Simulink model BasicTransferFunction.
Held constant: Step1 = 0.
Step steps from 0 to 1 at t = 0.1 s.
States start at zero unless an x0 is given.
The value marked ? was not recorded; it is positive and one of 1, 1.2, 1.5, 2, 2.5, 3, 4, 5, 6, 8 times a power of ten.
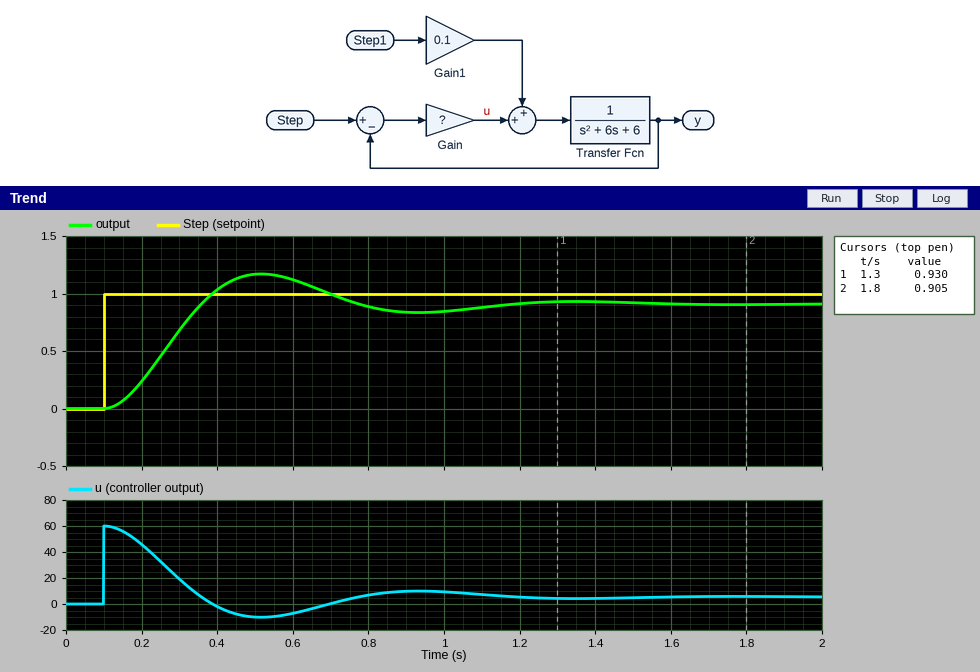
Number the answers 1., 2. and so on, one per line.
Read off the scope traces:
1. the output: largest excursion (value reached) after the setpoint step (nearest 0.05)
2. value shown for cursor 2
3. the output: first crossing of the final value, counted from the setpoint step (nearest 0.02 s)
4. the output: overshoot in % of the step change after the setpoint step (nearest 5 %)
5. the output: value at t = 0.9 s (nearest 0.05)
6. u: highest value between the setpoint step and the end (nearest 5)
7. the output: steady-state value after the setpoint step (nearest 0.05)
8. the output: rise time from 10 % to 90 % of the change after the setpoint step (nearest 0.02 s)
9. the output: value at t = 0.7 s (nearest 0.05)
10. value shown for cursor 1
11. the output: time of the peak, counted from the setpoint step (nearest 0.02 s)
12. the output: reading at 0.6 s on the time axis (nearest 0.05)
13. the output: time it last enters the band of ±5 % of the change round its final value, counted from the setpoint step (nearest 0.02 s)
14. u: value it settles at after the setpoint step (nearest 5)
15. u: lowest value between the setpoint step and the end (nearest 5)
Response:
1. 1.15
2. 0.905
3. 0.26 s
4. 30 %
5. 0.85
6. 60
7. 0.90
8. 0.18 s
9. 1.00
10. 0.930
11. 0.42 s
12. 1.10
13. 0.96 s
14. 5
15. -10
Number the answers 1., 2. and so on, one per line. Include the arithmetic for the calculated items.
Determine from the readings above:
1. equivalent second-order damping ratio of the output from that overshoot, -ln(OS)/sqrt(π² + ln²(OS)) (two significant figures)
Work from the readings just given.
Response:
1. ln(0.3) = -1.204; 1.204 / sqrt(9.870 + 1.450) = 0.36
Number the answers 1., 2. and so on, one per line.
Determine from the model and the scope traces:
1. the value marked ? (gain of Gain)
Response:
1. 60
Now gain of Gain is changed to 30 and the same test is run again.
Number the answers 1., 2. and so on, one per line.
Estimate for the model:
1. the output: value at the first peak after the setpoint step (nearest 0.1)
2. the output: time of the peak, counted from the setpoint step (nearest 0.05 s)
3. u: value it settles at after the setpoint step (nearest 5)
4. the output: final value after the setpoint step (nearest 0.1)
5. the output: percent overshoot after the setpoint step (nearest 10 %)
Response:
1. 1.0
2. 0.60 s
3. 5
4. 0.8
5. 20 %
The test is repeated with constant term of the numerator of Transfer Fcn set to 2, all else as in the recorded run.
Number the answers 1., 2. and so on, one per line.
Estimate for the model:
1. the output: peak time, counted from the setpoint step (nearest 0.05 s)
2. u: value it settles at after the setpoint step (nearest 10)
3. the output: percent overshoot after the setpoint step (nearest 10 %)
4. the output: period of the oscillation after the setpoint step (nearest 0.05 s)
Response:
1. 0.30 s
2. 0
3. 40 %
4. 0.60 s
